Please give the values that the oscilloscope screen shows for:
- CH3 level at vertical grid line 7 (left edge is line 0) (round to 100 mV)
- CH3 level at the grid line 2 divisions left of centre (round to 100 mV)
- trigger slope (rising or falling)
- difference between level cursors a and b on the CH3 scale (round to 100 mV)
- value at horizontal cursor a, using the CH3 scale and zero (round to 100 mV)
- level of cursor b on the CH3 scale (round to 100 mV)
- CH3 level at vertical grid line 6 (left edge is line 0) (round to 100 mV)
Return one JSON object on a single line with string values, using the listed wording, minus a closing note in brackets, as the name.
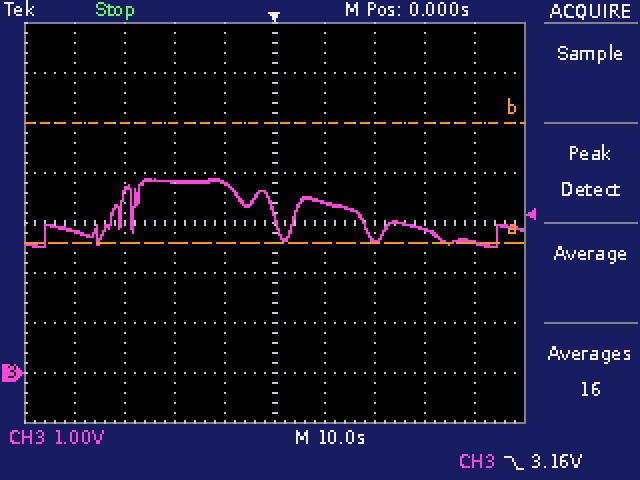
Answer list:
{"CH3 level at vertical grid line 7 (left edge is line 0)": "2.7 V", "CH3 level at the grid line 2 divisions left of centre": "3.8 V", "trigger slope": "falling", "difference between level cursors a and b on the CH3 scale": "2.4 V", "value at horizontal cursor a, using the CH3 scale and zero": "2.6 V", "level of cursor b on the CH3 scale": "5.0 V", "CH3 level at vertical grid line 6 (left edge is line 0)": "3.4 V"}
